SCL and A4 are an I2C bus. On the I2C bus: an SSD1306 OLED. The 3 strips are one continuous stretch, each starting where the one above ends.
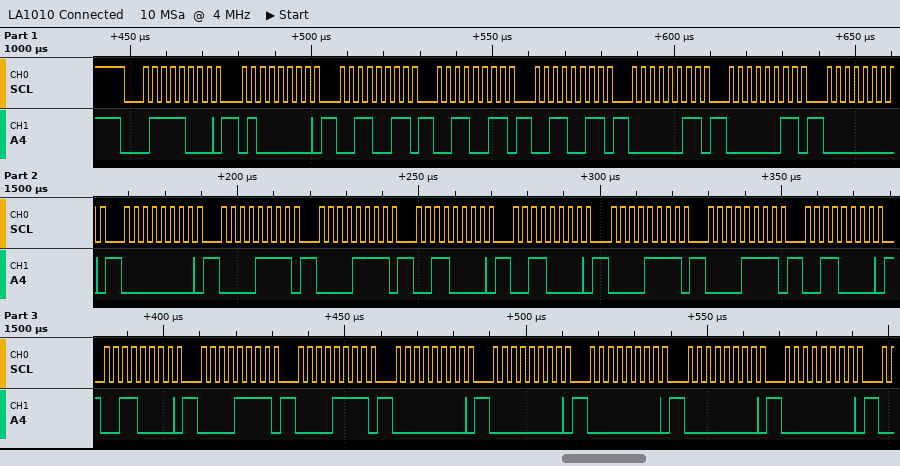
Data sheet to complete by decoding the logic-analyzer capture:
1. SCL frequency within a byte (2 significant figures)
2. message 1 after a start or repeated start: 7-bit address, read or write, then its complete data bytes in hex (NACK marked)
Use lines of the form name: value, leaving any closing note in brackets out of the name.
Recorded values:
SCL frequency within a byte: 400 kHz
message 1 after a start or repeated start: 7-bit address, read or write, then its complete data bytes in hex: 0x3C write: 40 33 33 33 03 03 00 00 0F 0F 30 30 0F 0F 30 30 0F 0F 00 00 00 00 00
